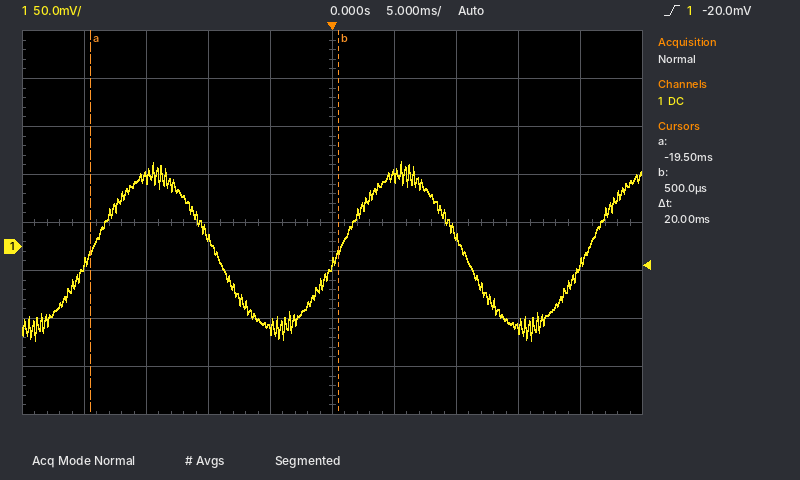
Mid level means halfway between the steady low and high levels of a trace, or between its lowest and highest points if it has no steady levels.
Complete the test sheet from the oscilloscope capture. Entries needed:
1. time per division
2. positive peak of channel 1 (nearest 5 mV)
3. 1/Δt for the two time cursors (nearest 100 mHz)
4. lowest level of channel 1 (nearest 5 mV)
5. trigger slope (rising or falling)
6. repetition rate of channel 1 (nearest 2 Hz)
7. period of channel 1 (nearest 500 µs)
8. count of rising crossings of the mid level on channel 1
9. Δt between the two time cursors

5 ms
90 mV
50.0 Hz
-100 mV
rising
50 Hz
20.0 ms
3
20 ms
